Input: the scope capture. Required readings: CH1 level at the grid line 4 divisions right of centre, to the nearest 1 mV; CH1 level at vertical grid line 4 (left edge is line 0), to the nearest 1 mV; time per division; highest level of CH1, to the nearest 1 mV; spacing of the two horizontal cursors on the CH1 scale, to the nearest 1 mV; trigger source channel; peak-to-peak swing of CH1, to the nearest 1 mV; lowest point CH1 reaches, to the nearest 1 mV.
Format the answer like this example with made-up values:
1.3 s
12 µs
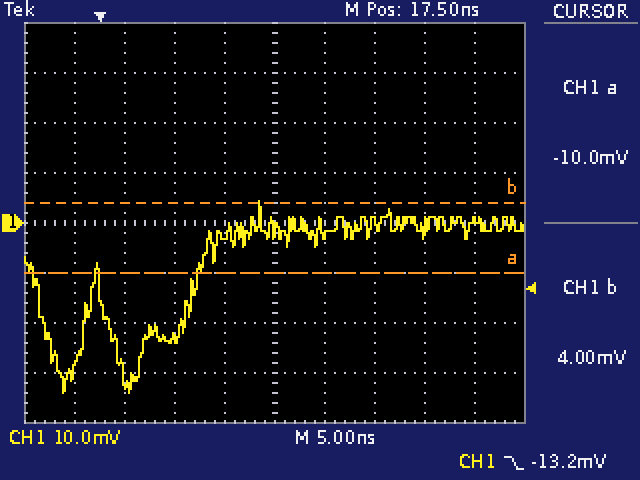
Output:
1 mV
-2 mV
5 ns
4 mV
14 mV
CH1
38 mV
-34 mV
